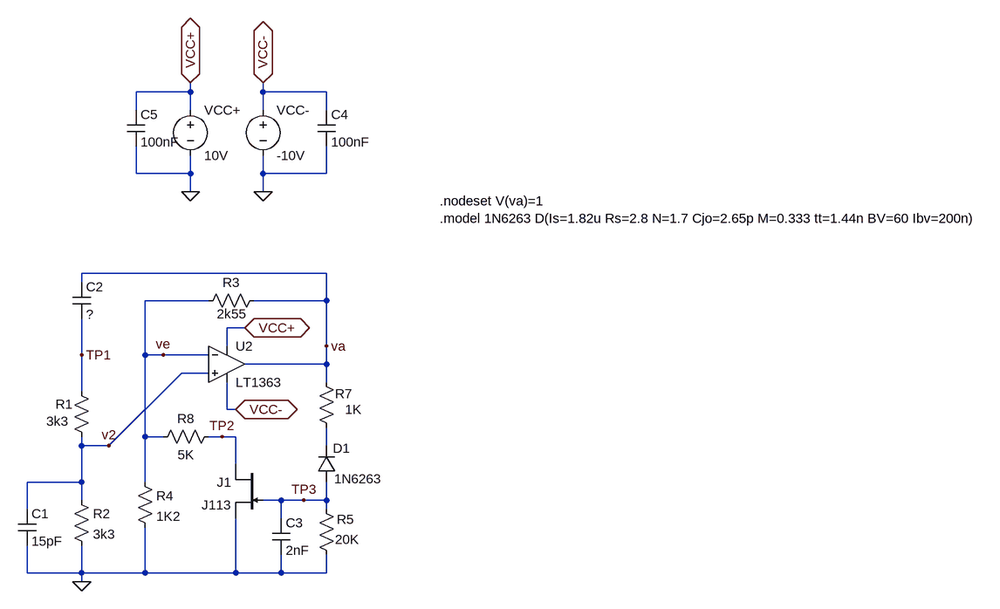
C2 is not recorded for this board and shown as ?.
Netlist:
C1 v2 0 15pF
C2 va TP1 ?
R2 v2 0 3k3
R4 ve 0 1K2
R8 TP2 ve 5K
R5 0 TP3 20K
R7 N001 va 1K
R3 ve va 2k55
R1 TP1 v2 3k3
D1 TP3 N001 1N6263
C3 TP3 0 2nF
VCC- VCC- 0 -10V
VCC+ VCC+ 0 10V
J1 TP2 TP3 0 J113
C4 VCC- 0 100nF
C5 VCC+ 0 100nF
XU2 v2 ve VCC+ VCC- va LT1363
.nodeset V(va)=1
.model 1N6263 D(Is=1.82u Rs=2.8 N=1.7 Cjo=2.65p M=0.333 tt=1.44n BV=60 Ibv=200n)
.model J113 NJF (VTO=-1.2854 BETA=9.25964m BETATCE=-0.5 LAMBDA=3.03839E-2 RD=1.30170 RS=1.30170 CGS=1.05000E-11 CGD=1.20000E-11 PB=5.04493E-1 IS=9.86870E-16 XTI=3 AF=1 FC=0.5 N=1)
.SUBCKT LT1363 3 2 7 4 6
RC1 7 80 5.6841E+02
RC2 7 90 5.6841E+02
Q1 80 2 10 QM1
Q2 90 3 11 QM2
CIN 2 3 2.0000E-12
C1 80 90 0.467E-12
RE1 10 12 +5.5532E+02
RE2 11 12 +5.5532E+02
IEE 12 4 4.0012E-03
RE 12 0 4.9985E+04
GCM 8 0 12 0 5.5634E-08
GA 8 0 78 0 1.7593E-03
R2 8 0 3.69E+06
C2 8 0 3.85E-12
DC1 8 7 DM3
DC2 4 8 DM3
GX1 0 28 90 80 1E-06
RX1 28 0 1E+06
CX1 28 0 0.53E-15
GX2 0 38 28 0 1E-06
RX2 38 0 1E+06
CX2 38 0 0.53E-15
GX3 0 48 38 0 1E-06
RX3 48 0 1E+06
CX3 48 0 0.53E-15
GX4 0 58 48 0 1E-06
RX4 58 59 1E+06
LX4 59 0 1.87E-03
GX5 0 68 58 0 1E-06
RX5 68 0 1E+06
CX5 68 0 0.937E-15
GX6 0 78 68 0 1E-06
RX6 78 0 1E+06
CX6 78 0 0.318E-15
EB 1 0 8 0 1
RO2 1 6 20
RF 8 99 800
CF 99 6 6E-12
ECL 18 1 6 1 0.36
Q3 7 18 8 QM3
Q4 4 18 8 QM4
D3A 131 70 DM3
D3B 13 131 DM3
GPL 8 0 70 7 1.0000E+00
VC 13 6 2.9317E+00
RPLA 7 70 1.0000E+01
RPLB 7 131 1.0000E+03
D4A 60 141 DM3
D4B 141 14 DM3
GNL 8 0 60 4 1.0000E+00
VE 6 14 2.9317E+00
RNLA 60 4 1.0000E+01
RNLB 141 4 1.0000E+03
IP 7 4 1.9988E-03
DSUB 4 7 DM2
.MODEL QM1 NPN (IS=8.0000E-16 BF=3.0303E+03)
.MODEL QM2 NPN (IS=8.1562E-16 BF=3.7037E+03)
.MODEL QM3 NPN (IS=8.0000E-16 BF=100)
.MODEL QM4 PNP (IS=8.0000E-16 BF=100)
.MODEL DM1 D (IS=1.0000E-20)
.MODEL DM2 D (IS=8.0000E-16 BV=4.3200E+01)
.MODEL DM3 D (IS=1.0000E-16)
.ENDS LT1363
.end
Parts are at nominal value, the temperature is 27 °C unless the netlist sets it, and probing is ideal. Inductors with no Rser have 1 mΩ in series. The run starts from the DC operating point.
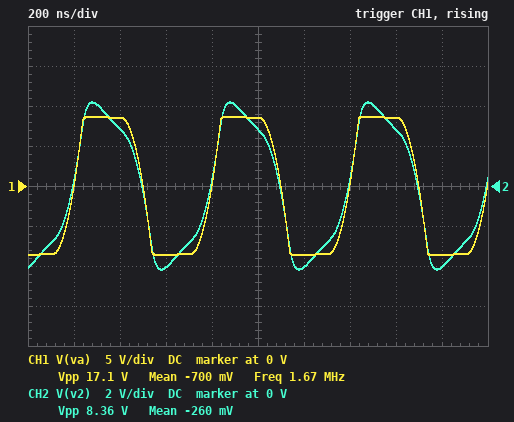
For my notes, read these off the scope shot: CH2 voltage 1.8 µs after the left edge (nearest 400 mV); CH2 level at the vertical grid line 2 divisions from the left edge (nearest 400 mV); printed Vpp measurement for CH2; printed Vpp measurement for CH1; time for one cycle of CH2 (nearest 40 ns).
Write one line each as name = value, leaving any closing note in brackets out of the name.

CH2 voltage 1.8 µs after the left edge = -4.0 V
CH2 level at the vertical grid line 2 divisions from the left edge = 2.8 V
printed Vpp measurement for CH2 = 8.36 V
printed Vpp measurement for CH1 = 17.1 V
time for one cycle of CH2 = 600 ns
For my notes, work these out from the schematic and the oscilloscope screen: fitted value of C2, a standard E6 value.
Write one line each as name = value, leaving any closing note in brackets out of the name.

fitted value of C2, a standard E6 value = 33 pF
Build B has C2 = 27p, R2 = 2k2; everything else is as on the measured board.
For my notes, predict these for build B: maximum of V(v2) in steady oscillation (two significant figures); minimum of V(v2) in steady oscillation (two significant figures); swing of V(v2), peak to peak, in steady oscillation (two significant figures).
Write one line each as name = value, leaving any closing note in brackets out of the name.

maximum of V(v2) in steady oscillation = 3.0 V
minimum of V(v2) in steady oscillation = -3.0 V
swing of V(v2), peak to peak, in steady oscillation = 6.0 V
